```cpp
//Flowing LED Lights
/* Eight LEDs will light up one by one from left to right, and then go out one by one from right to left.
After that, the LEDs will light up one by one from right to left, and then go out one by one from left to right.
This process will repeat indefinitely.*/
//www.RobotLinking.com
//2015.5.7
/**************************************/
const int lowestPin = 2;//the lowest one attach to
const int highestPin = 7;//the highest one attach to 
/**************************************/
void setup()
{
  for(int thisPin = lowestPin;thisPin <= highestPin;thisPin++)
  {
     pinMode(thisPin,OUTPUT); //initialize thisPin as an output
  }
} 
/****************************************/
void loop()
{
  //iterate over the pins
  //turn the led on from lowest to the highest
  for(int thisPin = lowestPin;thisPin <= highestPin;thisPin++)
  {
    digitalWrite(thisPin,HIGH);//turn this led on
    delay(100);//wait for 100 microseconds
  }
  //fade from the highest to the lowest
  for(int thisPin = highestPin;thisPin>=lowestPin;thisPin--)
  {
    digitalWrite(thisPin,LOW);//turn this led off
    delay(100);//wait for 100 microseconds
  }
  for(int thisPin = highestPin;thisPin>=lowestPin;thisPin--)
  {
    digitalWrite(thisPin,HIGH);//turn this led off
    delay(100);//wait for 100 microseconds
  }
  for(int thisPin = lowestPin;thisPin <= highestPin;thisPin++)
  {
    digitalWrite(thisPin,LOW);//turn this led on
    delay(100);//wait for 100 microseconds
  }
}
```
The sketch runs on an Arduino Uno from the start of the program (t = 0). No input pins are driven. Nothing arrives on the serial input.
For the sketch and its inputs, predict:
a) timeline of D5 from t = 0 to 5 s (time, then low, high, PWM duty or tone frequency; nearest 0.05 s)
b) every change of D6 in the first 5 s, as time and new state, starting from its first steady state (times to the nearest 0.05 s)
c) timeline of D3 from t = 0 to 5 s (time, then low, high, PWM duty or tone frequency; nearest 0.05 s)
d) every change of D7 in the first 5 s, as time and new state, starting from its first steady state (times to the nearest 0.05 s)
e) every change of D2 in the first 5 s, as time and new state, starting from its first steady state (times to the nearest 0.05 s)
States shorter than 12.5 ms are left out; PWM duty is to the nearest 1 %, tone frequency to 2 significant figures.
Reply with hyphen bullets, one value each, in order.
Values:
- 0 s low; 0.3 s high; 0.8 s low; 1.4 s high; 2.1 s low; 2.7 s high; 3.2 s low; 3.8 s high; 4.5 s low
- 0 s low; 0.4 s high; 0.7 s low; 1.3 s high; 2.2 s low; 2.8 s high; 3.1 s low; 3.7 s high; 4.6 s low
- 0 s low; 0.1 s high; 1 s low; 1.6 s high; 1.9 s low; 2.5 s high; 3.4 s low; 4 s high; 4.3 s low; 4.9 s high
- 0 s low; 0.5 s high; 0.6 s low; 1.2 s high; 2.3 s low; 2.9 s high; 3 s low; 3.6 s high; 4.7 s low
- 0 s high; 1.1 s low; 1.7 s high; 1.8 s low; 2.4 s high; 3.5 s low; 4.1 s high; 4.2 s low; 4.8 s high
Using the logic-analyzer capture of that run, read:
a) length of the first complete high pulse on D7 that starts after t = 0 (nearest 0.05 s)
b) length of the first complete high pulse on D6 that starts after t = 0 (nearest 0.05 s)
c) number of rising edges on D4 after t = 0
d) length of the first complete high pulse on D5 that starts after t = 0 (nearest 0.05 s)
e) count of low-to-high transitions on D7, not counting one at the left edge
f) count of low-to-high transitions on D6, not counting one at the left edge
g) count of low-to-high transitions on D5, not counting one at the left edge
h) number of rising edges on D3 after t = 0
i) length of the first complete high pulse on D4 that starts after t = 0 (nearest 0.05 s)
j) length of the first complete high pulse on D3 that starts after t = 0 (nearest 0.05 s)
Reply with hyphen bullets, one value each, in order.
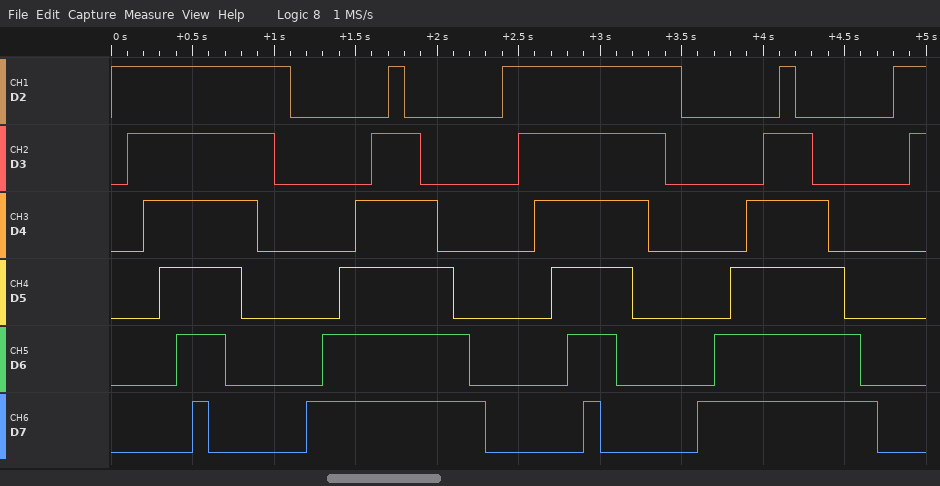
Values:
- 0.10 s
- 0.30 s
- 4
- 0.50 s
- 4
- 4
- 4
- 5
- 0.70 s
- 0.90 s
